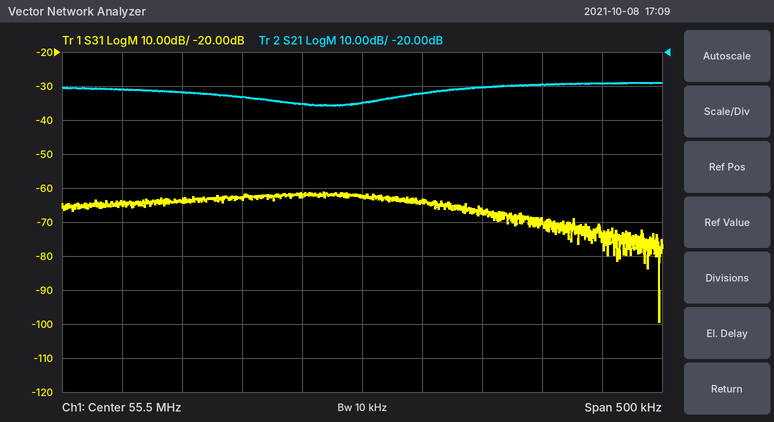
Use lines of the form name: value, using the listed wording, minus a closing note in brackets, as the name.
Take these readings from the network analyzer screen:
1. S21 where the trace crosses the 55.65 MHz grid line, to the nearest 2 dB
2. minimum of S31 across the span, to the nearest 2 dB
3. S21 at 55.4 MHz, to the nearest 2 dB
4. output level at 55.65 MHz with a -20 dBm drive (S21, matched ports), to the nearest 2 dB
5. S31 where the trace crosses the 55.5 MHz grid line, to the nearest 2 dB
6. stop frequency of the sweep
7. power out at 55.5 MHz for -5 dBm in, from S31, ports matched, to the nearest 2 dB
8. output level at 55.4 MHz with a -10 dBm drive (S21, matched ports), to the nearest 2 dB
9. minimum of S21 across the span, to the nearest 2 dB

S21 where the trace crosses the 55.65 MHz grid line, to the nearest 2 dB: -30 dB
minimum of S31 across the span, to the nearest 2 dB: -100 dB
S21 at 55.4 MHz, to the nearest 2 dB: -34 dB
output level at 55.65 MHz with a -20 dBm drive (S21, matched ports), to the nearest 2 dB: -50 dBm
S31 where the trace crosses the 55.5 MHz grid line, to the nearest 2 dB: -62 dB
stop frequency of the sweep: 55.75 MHz
power out at 55.5 MHz for -5 dBm in, from S31, ports matched, to the nearest 2 dB: -68 dBm
output level at 55.4 MHz with a -10 dBm drive (S21, matched ports), to the nearest 2 dB: -44 dBm
minimum of S21 across the span, to the nearest 2 dB: -36 dB
